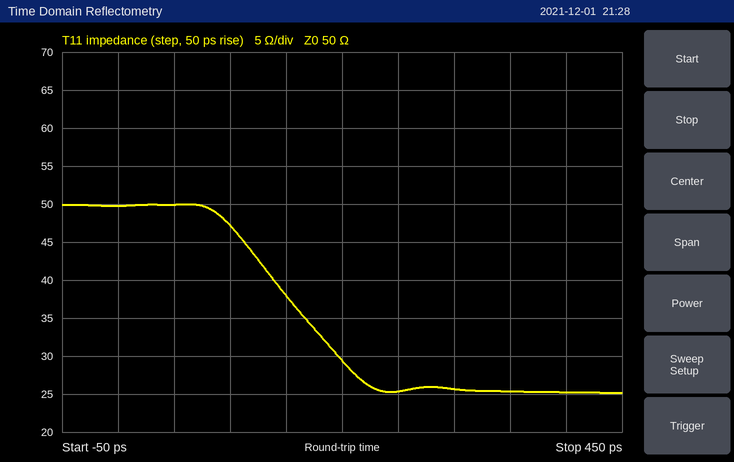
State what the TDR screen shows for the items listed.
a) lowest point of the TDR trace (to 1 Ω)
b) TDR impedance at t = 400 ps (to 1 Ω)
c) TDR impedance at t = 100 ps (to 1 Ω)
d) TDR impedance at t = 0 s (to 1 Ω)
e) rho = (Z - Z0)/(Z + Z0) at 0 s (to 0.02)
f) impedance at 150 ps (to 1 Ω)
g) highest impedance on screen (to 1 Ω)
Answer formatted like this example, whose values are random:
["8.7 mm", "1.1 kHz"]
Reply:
["25 Ω", "25 Ω", "47 Ω", "50 Ω", "0.00", "38 Ω", "50 Ω"]
